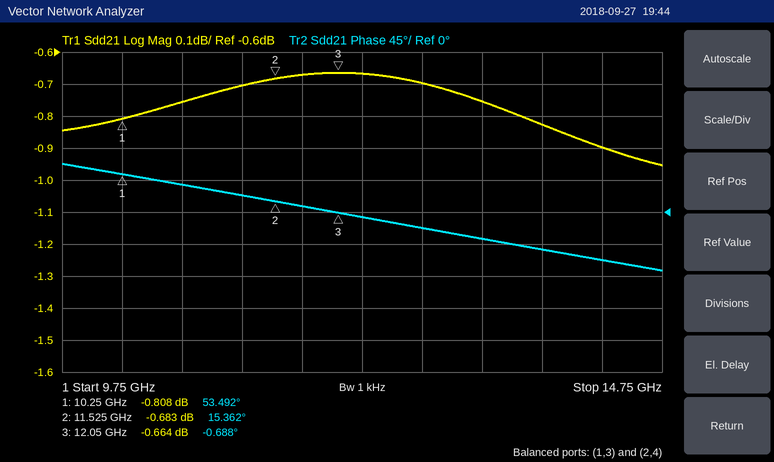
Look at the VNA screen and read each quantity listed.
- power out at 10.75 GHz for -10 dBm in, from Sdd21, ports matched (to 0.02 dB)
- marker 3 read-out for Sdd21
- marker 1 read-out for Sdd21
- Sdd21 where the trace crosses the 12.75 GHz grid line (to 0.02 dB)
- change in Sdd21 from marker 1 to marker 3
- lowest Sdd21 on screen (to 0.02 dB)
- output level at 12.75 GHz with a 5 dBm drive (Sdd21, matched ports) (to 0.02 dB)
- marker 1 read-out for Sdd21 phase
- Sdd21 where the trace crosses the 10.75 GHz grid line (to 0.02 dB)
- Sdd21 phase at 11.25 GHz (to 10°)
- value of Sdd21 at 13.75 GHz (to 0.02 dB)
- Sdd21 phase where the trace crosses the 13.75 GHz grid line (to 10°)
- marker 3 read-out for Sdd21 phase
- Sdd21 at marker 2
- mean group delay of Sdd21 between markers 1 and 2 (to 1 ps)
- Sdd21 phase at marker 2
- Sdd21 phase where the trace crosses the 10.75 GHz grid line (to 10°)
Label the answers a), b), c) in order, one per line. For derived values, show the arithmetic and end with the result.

a) -10 dBm + (-0.76 dB) = -10.76 dBm
b) -0.664 dB
c) -0.808 dB
d) -0.70 dB
e) -0.664 − (-0.808) = 0.144 dB
f) -0.96 dB
g) 5 dBm + (-0.70 dB) = 4.30 dBm
h) 53.492°
i) -0.76 dB
j) 20°
k) -0.82 dB
l) -50°
m) -0.688°
n) -0.683 dB
o) −(15.362° − (53.492°))/(360° × 1.275 GHz) ≈ 83 ps
p) 15.362°
q) 40°
